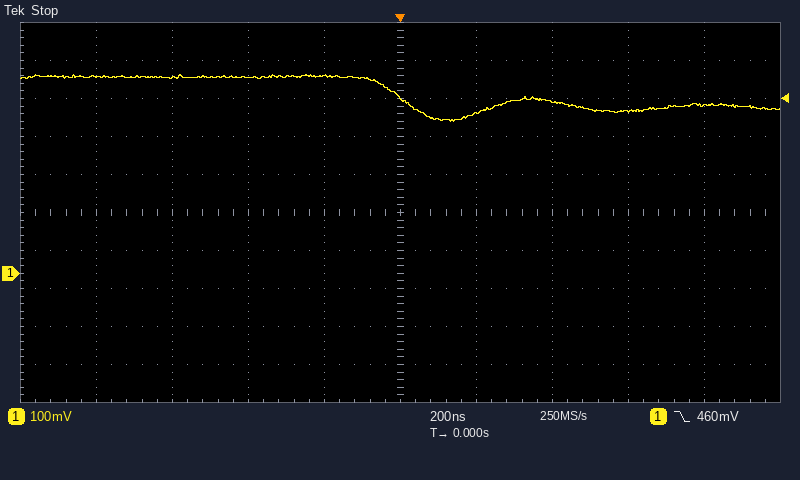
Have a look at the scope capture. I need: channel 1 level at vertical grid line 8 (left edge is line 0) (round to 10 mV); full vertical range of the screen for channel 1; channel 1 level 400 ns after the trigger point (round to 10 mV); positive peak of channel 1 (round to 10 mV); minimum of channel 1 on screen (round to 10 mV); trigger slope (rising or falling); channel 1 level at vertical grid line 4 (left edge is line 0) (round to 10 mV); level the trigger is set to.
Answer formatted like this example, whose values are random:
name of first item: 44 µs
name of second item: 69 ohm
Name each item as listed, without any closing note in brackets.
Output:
channel 1 level at vertical grid line 8 (left edge is line 0): 430 mV
full vertical range of the screen for channel 1: 1 V
channel 1 level 400 ns after the trigger point: 450 mV
positive peak of channel 1: 520 mV
minimum of channel 1 on screen: 400 mV
trigger slope: falling
channel 1 level at vertical grid line 4 (left edge is line 0): 520 mV
level the trigger is set to: 460 mV
